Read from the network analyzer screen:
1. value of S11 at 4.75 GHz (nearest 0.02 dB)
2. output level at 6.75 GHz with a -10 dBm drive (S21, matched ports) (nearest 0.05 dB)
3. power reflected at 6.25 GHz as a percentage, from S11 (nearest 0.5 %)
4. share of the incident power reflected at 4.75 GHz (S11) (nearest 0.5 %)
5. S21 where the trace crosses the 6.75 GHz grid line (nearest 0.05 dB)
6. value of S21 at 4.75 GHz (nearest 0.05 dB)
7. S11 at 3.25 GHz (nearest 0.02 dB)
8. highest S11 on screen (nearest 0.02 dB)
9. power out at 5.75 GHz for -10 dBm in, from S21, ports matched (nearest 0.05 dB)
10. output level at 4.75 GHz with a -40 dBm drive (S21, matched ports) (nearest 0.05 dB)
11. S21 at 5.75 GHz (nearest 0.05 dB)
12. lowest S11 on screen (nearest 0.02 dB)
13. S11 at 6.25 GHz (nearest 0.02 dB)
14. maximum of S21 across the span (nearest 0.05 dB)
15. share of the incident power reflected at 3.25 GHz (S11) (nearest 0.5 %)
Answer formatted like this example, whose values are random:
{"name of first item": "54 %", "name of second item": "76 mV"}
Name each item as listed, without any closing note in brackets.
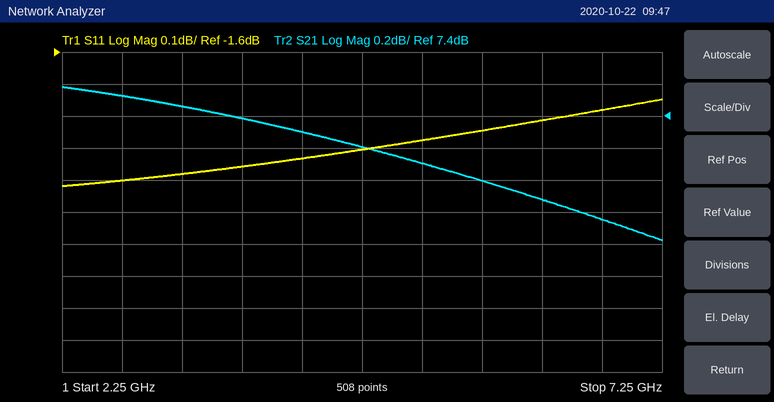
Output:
{"value of S11 at 4.75 GHz": "-1.90 dB", "output level at 6.75 GHz with a -10 dBm drive (S21, matched ports)": "-3.25 dBm", "power reflected at 6.25 GHz as a percentage, from S11": "66.0 %", "share of the incident power reflected at 4.75 GHz (S11)": "64.5 %", "S21 where the trace crosses the 6.75 GHz grid line": "6.75 dB", "value of S21 at 4.75 GHz": "7.20 dB", "S11 at 3.25 GHz": "-1.98 dB", "highest S11 on screen": "-1.74 dB", "power out at 5.75 GHz for -10 dBm in, from S21, ports matched": "-3.00 dBm", "output level at 4.75 GHz with a -40 dBm drive (S21, matched ports)": "-32.80 dBm", "S21 at 5.75 GHz": "7.00 dB", "lowest S11 on screen": "-2.02 dB", "S11 at 6.25 GHz": "-1.82 dB", "maximum of S21 across the span": "7.60 dB", "share of the incident power reflected at 3.25 GHz (S11)": "63.5 %"}
